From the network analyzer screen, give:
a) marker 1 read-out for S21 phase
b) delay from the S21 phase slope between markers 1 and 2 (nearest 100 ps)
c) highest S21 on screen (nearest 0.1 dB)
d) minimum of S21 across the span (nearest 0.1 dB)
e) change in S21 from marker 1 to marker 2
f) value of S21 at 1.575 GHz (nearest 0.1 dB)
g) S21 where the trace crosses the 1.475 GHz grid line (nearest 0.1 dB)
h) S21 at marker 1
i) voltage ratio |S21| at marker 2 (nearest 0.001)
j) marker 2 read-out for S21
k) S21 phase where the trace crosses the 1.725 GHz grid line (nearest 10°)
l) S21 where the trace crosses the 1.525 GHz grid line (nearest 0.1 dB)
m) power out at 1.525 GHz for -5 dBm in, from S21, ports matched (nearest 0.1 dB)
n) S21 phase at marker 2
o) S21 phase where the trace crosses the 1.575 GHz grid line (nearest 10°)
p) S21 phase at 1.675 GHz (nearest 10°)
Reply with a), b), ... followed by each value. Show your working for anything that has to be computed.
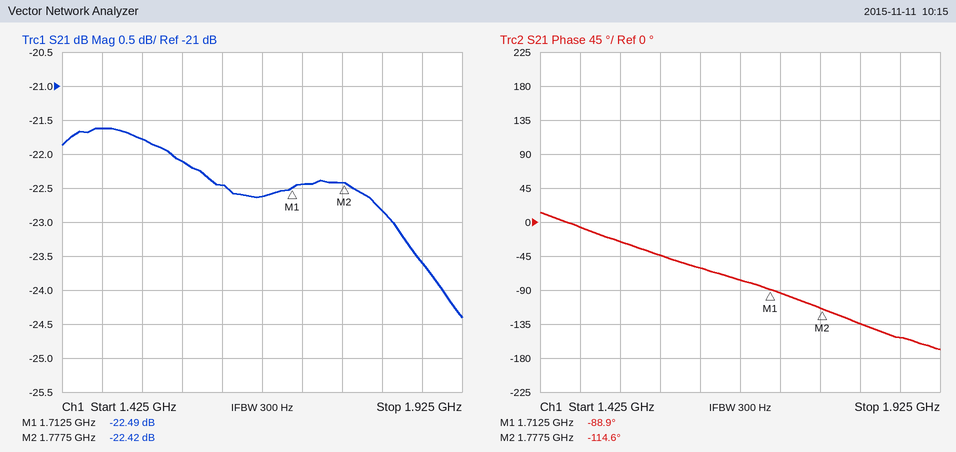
a) -88.9°
b) −(-114.6° − (-88.9°))/(360° × 65 MHz) ≈ 1.1 ns
c) -21.6 dB
d) -24.4 dB
e) -22.42 − (-22.49) = 0.07 dB
f) -22.1 dB
g) -21.6 dB
h) -22.49 dB
i) 10^(-22.42/20) ≈ 0.076
j) -22.42 dB
k) -90°
l) -21.8 dB
m) -5 dBm + (-21.8 dB) = -26.8 dBm
n) -114.6°
o) -40°
p) -80°
